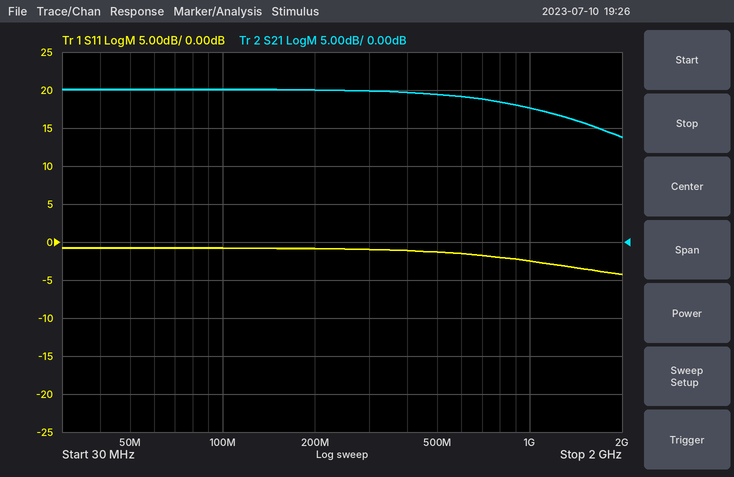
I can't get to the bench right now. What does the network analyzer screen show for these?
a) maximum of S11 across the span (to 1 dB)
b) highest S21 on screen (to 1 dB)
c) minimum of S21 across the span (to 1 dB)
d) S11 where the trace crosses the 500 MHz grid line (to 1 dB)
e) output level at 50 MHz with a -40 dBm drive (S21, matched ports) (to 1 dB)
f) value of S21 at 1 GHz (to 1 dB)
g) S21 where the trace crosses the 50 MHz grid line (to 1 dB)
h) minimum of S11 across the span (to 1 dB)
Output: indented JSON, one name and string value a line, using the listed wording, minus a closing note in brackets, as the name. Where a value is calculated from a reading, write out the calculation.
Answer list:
{
  "maximum of S11 across the span": "-1 dB",
  "highest S21 on screen": "20 dB",
  "minimum of S21 across the span": "14 dB",
  "S11 where the trace crosses the 500 MHz grid line": "-1 dB",
  "output level at 50 MHz with a -40 dBm drive (S21, matched ports)": "-40 dBm + (20 dB) = -20 dBm",
  "value of S21 at 1 GHz": "18 dB",
  "S21 where the trace crosses the 50 MHz grid line": "20 dB",
  "minimum of S11 across the span": "-4 dB"
}
